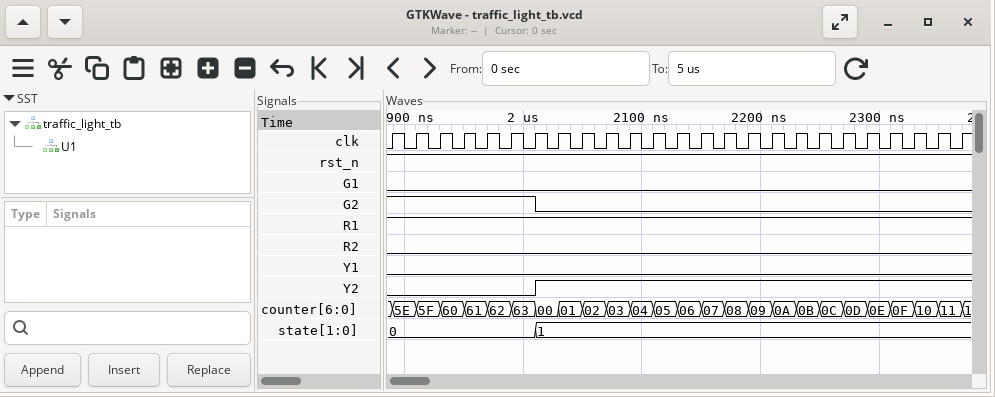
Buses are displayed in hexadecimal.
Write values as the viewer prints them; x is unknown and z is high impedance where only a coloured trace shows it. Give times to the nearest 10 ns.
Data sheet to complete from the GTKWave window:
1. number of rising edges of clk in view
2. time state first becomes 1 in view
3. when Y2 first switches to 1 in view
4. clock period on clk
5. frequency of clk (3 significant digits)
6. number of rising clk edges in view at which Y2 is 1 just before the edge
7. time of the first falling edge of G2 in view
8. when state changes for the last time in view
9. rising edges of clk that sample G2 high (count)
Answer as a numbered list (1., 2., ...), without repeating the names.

1. 25
2. 2010 ns
3. 2010 ns
4. 20 ns
5. 50.0 MHz
6. 18
7. 2010 ns
8. 2010 ns
9. 7
